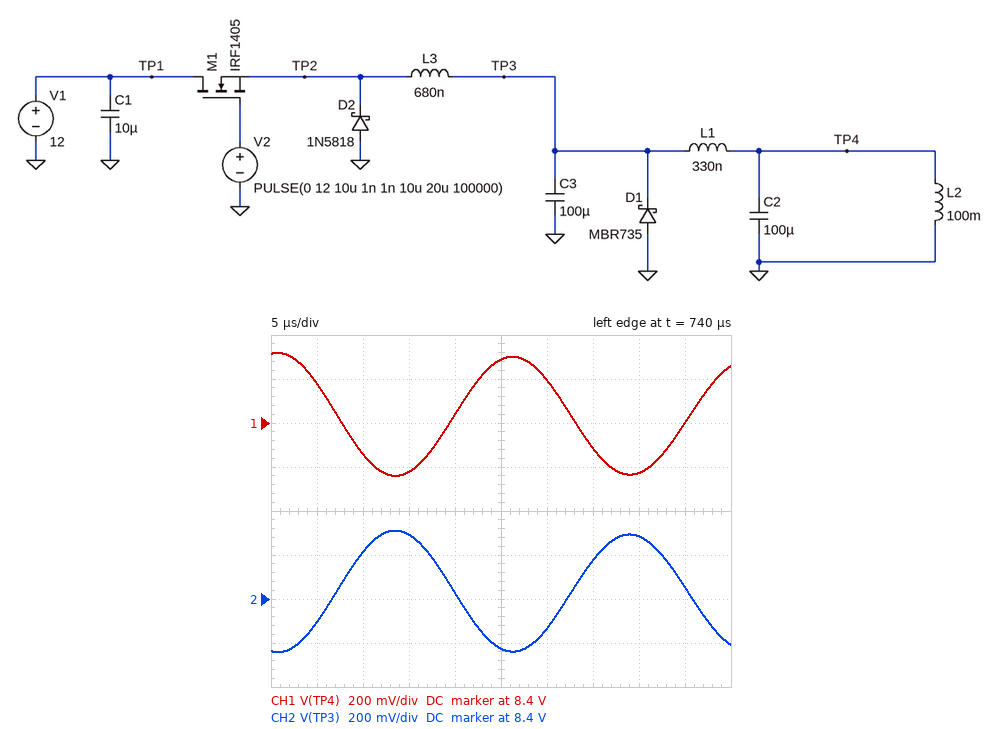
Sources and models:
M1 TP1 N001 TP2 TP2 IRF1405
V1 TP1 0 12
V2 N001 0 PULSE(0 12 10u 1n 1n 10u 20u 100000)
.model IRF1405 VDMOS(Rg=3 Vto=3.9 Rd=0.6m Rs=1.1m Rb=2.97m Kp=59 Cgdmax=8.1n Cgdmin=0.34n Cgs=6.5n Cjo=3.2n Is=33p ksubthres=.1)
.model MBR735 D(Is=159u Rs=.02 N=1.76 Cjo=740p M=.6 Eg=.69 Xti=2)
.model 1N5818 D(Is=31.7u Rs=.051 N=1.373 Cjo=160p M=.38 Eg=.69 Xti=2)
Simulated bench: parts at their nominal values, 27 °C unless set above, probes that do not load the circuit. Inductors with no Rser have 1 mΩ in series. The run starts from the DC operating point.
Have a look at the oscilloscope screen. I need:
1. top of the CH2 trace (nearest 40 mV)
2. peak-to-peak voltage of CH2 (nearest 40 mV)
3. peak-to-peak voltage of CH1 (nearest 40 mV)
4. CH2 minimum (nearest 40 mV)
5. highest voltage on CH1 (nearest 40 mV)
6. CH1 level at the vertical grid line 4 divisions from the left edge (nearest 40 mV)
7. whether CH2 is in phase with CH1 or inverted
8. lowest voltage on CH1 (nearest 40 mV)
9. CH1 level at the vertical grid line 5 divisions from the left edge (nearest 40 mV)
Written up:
8.72 V
560 mV
560 mV
8.16 V
8.72 V
8.44 V
inverted
8.16 V
8.68 V
